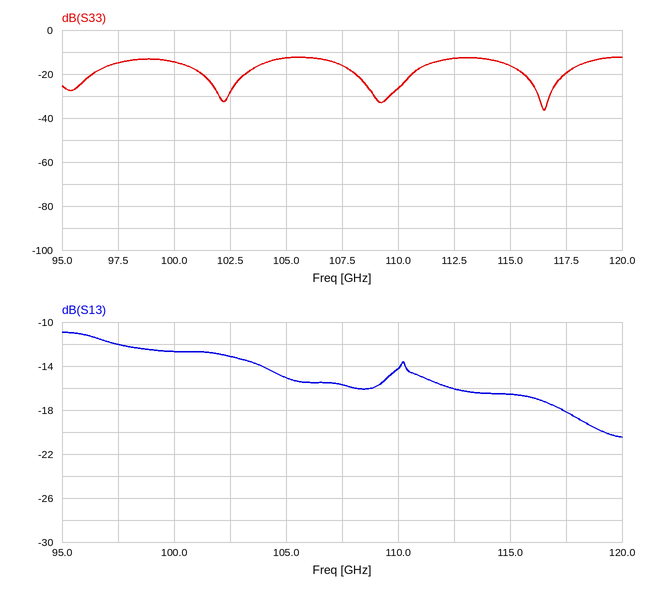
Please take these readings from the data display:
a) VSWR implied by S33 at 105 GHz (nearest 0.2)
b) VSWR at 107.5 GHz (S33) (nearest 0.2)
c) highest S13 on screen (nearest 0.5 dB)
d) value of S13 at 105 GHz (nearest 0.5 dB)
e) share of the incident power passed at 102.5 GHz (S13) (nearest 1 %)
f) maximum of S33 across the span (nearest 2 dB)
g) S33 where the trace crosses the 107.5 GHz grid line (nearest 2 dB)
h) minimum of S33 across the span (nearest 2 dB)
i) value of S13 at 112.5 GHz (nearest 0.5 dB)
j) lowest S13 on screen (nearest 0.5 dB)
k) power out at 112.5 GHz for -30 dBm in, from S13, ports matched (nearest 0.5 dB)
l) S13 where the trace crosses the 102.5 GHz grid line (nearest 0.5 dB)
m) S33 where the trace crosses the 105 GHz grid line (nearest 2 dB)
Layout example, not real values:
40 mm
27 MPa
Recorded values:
1.6
1.4
-11.0 dB
-15.0 dB
5 %
-12 dB
-16 dB
-36 dB
-16.0 dB
-20.5 dB
-46.0 dBm
-13.0 dB
-12 dB
